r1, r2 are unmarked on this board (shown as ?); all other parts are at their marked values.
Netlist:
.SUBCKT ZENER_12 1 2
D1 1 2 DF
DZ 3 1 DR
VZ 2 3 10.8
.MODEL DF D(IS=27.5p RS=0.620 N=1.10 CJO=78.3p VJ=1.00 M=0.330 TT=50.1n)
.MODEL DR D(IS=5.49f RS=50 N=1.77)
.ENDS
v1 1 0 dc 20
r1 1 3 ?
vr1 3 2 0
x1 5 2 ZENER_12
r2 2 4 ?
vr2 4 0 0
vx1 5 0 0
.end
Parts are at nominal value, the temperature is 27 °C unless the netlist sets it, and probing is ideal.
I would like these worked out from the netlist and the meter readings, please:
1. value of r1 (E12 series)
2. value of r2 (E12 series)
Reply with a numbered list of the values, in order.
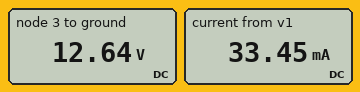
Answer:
1. 220 Ω
2. 560 Ω
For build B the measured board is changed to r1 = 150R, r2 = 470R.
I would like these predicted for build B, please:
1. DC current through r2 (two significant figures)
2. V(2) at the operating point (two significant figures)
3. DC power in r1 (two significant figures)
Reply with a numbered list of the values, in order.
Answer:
1. 28 mA
2. 13 V
3. 320 mW
